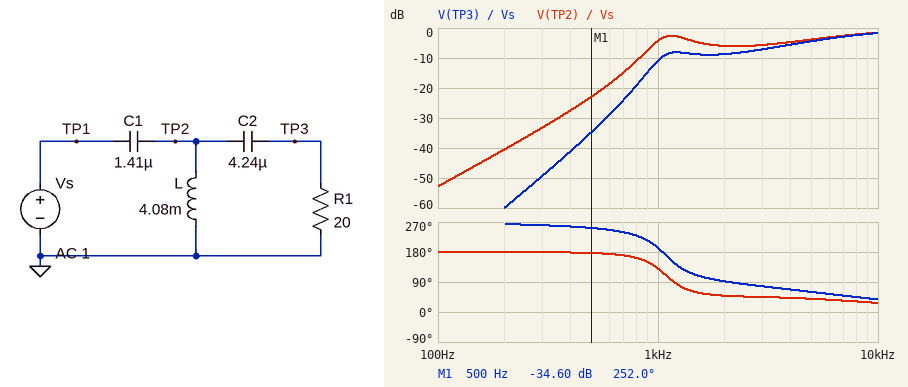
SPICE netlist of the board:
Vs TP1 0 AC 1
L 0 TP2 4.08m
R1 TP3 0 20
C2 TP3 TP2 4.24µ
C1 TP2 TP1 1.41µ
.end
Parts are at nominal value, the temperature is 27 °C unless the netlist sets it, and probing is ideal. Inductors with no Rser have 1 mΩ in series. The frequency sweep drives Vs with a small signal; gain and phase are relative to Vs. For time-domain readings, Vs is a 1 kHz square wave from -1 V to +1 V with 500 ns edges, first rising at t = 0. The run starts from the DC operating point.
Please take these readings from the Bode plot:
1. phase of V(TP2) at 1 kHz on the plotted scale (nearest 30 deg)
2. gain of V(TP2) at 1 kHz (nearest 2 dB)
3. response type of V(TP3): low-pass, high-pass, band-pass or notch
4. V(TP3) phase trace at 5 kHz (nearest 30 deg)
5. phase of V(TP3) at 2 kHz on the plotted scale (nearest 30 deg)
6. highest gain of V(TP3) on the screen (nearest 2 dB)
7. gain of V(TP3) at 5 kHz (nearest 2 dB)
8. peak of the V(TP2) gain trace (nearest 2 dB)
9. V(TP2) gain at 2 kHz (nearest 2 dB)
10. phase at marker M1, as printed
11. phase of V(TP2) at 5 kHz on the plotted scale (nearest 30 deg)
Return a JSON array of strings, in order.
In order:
["120 deg", "-4 dB", "high-pass", "60 deg", "90 deg", "-2 dB", "-4 dB", "-2 dB", "-6 dB", "252.0 deg", "30 deg"]
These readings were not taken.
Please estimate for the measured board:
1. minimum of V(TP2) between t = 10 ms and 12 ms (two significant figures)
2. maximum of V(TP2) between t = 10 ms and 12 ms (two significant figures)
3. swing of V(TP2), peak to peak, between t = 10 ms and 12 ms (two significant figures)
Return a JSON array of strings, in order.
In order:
["-2.3 V", "2.3 V", "4.6 V"]
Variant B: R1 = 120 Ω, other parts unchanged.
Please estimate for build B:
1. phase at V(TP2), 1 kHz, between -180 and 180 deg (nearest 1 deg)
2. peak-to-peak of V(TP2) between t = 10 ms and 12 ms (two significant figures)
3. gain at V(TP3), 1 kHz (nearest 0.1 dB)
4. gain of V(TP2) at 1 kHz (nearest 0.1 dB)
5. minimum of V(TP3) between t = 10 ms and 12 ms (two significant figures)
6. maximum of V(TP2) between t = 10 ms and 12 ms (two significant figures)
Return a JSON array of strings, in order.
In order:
["165 deg", "3.2 V", "-10.6 dB", "-10.2 dB", "-1.6 V", "1.6 V"]
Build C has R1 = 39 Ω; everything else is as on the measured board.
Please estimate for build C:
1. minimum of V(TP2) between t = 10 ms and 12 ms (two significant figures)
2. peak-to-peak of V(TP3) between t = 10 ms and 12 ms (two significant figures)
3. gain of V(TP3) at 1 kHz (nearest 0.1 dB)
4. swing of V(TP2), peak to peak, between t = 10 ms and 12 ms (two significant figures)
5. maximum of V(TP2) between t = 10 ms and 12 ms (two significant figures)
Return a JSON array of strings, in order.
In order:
["-2.0 V", "3.6 V", "-10.7 dB", "4.0 V", "2.0 V"]
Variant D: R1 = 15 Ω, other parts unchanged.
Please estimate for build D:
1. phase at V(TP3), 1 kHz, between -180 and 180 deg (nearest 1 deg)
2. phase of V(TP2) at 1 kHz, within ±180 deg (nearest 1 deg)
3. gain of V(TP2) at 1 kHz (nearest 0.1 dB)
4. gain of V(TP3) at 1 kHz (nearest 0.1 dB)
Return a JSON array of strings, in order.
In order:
["-164 deg", "128 deg", "-2.4 dB", "-11.0 dB"]
